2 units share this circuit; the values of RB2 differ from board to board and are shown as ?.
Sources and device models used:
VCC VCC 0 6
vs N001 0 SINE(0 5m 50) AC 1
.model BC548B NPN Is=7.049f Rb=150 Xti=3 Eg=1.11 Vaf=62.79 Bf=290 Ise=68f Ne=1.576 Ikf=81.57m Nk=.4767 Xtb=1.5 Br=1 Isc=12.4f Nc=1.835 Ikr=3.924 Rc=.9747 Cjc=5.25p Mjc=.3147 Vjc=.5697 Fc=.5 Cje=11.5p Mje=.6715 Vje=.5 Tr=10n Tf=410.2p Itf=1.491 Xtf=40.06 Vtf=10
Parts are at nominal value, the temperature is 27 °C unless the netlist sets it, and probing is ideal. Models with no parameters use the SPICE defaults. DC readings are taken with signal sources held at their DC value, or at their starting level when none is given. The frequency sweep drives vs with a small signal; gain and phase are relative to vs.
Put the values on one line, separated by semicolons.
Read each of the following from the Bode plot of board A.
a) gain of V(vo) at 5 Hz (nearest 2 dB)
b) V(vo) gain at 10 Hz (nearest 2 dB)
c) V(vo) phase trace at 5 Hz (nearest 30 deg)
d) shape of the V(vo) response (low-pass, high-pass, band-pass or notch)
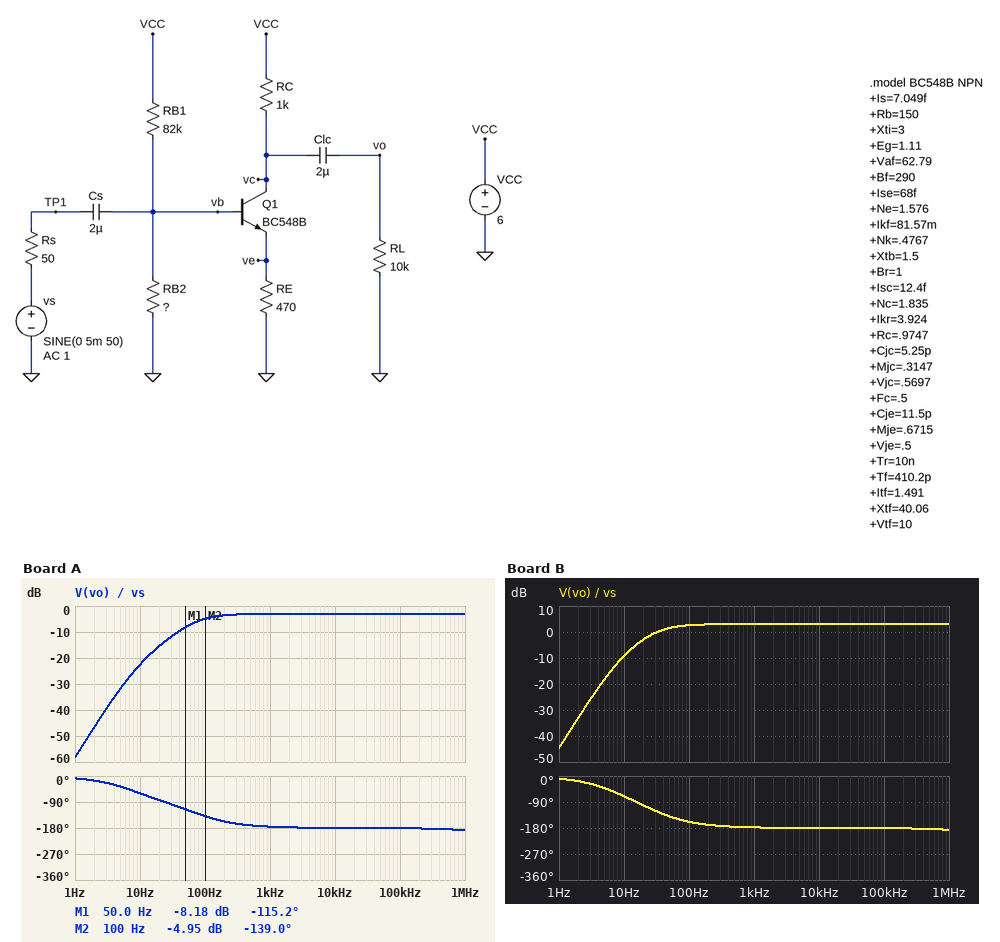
-32 dB; -22 dB; -30 deg; high-pass
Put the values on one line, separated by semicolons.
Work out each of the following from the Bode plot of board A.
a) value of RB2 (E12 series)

270 kΩ
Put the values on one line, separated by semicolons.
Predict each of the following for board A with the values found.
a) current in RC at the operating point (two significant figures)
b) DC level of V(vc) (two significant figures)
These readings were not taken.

4.0 mA; 2.0 V
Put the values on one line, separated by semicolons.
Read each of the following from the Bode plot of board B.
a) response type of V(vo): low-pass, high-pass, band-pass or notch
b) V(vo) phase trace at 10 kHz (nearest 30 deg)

high-pass; -180 deg
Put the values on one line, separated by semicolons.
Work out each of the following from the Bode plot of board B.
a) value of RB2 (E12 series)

120 kΩ
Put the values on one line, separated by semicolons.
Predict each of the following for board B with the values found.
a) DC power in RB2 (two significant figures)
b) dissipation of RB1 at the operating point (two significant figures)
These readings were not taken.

55 µW; 140 µW
